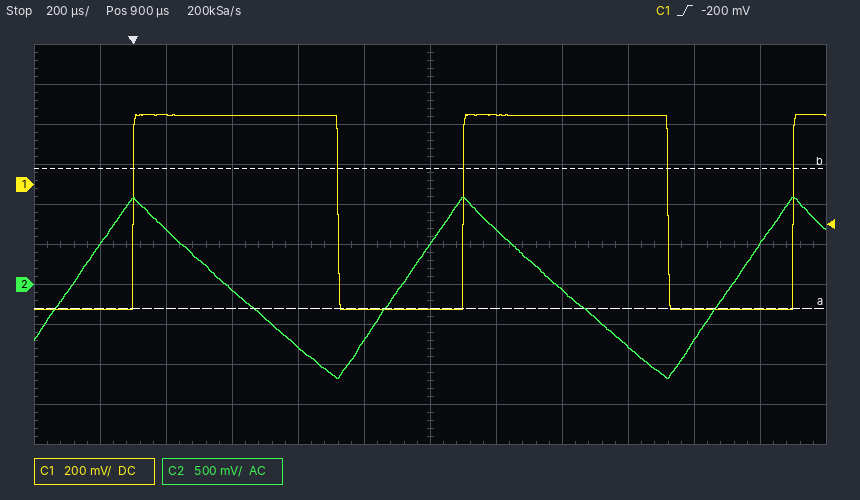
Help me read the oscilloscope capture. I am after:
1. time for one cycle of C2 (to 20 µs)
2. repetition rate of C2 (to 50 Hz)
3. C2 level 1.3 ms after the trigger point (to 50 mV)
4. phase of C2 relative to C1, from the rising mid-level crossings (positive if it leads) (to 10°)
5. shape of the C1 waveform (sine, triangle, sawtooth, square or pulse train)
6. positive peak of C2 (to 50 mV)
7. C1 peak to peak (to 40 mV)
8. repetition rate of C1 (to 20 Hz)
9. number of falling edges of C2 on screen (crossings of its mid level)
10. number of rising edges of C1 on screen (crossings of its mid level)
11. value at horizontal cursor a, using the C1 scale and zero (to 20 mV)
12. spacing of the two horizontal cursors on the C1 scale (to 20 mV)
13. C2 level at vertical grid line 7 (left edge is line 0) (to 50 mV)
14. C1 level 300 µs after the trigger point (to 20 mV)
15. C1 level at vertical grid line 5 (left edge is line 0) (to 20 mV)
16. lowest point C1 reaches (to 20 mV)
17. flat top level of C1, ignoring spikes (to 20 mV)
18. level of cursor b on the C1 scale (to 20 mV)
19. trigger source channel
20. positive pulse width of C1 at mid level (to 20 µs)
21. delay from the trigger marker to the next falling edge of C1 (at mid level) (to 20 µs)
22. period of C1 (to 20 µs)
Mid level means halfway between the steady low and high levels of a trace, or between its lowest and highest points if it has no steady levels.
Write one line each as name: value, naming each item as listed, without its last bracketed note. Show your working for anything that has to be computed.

time for one cycle of C2: 1.00 ms
repetition rate of C2: 1 / 1.00 ms ≈ 1.00 kHz
C2 level 1.3 ms after the trigger point: -50 mV
phase of C2 relative to C1, from the rising mid-level crossings (positive if it leads): +70°
shape of the C1 waveform: pulse train
positive peak of C2: 1.10 V
C1 peak to peak: 960 mV
repetition rate of C1: 1 / 1.00 ms ≈ 1.00 kHz
number of falling edges of C2 on screen: 2
number of rising edges of C1 on screen: 3
value at horizontal cursor a, using the C1 scale and zero: -620 mV
spacing of the two horizontal cursors on the C1 scale: 700 mV
C2 level at vertical grid line 7 (left edge is line 0): 700 mV
C1 level 300 µs after the trigger point: 340 mV
C1 level at vertical grid line 5 (left edge is line 0): -620 mV
lowest point C1 reaches: -620 mV
flat top level of C1, ignoring spikes: 340 mV
level of cursor b on the C1 scale: 80 mV
trigger source channel: C1
positive pulse width of C1 at mid level: 620 µs
delay from the trigger marker to the next falling edge of C1 (at mid level): 620 µs
period of C1: 1.00 ms
